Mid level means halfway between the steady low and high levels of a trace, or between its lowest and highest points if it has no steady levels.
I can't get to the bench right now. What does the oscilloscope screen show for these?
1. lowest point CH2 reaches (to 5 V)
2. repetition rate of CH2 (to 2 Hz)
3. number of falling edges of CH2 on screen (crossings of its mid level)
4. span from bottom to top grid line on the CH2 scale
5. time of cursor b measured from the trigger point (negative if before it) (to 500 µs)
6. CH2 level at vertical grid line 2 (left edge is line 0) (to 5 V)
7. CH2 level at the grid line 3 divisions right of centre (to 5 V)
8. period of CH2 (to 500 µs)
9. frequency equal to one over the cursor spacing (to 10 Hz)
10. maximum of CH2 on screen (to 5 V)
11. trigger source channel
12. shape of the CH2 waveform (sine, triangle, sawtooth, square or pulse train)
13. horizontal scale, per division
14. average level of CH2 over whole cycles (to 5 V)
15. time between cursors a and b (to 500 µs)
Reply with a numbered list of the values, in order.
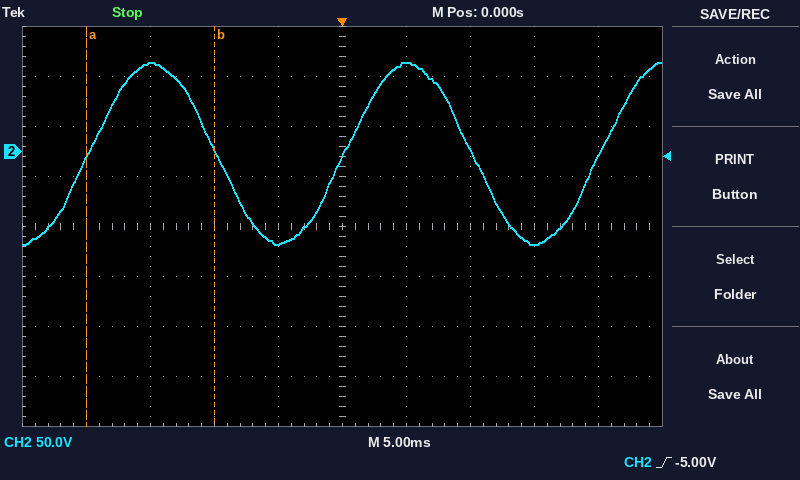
1. -95 V
2. 50 Hz
3. 2
4. 400 V
5. -10.0 ms
6. 90 V
7. -95 V
8. 20.0 ms
9. 100 Hz
10. 90 V
11. CH2
12. sine
13. 5 ms
14. 0 V
15. 10.0 ms
